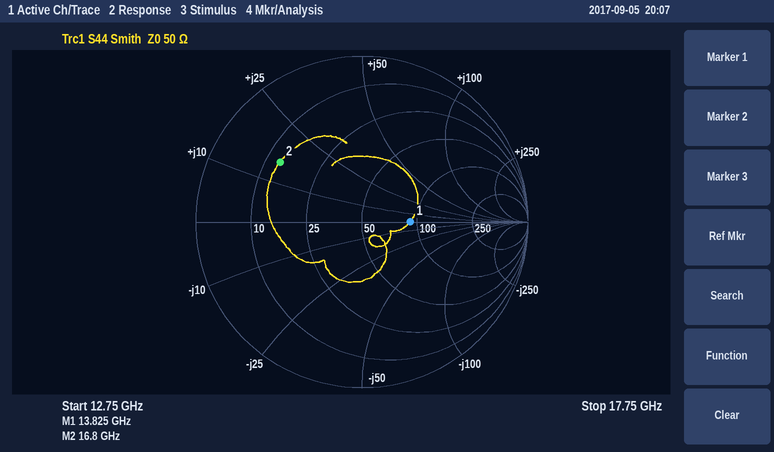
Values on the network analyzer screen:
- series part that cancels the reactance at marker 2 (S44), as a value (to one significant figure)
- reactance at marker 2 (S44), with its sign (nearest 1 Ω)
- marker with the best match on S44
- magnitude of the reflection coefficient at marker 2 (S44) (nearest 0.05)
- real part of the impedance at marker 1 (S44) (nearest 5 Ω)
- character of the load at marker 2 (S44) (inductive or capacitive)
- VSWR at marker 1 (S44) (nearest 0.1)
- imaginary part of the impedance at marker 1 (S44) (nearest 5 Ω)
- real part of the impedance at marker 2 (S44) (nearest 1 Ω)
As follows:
600 fF
+15 Ω
marker 1
0.60
90 Ω
inductive
1.8
0 Ω
13 Ω
